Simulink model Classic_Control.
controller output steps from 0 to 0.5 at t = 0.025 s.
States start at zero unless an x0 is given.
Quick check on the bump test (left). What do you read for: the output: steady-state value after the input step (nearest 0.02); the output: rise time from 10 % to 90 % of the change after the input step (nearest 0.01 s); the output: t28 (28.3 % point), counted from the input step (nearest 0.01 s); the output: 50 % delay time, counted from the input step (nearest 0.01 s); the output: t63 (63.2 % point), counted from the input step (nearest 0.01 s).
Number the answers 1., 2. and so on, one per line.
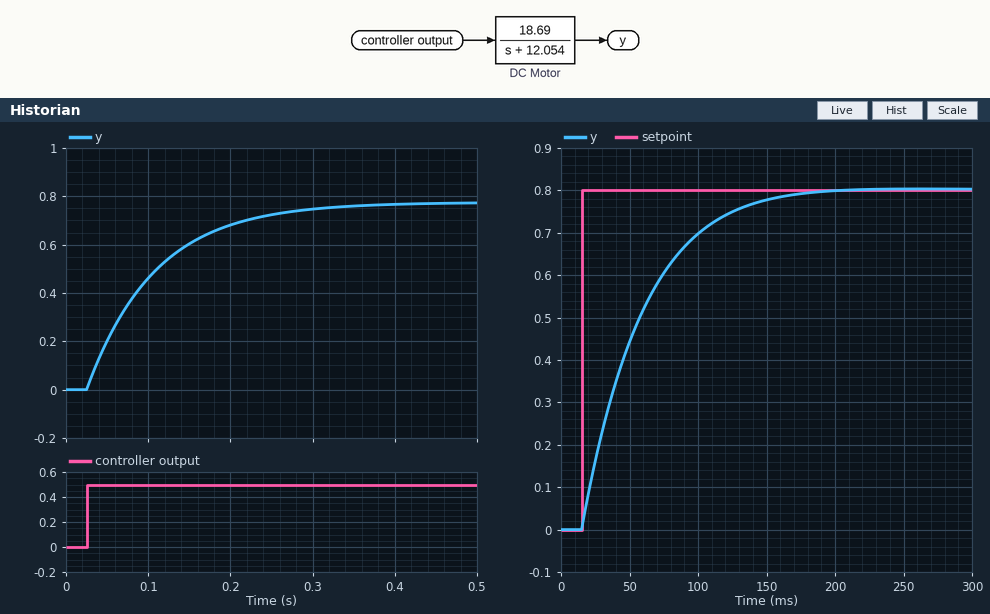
1. 0.78
2. 0.18 s
3. 0.03 s
4. 0.06 s
5. 0.08 s
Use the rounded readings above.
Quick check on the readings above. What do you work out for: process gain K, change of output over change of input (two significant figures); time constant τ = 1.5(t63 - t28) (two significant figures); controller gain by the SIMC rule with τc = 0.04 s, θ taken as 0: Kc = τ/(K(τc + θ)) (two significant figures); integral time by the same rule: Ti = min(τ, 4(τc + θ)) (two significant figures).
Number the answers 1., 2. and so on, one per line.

1. 1.6
2. 0.075 s
3. 1.2
4. 0.075 s
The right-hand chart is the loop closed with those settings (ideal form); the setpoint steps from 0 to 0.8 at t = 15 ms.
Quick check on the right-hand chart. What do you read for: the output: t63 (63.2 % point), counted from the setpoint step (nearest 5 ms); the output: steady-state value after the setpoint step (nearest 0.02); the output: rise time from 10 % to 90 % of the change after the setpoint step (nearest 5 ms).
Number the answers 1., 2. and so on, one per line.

1. 45 ms
2. 0.80
3. 90 ms
